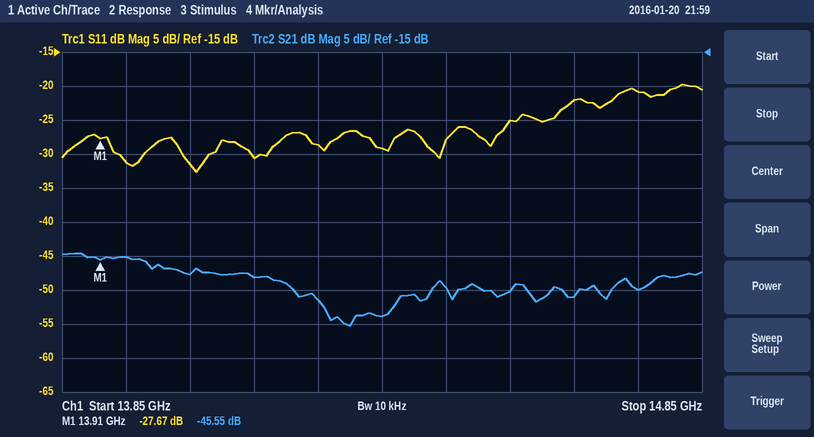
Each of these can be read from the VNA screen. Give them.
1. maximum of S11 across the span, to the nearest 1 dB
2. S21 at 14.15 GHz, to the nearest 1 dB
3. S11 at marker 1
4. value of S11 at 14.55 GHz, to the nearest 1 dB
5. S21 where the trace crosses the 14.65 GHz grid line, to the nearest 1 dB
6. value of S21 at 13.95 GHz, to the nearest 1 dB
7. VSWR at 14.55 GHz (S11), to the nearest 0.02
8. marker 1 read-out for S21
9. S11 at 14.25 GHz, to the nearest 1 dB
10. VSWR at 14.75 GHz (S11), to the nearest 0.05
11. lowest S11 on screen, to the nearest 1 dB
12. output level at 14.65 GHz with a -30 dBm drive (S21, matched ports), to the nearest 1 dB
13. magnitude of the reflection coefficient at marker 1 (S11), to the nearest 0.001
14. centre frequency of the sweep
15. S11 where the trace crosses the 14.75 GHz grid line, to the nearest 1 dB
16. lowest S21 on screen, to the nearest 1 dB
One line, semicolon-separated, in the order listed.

-20 dB; -48 dB; -27.67 dB; -25 dB; -51 dB; -45 dB; 1.12; -45.55 dB; -29 dB; 1.20; -33 dB; -81 dBm; 0.041; 14.35 GHz; -21 dB; -55 dB
